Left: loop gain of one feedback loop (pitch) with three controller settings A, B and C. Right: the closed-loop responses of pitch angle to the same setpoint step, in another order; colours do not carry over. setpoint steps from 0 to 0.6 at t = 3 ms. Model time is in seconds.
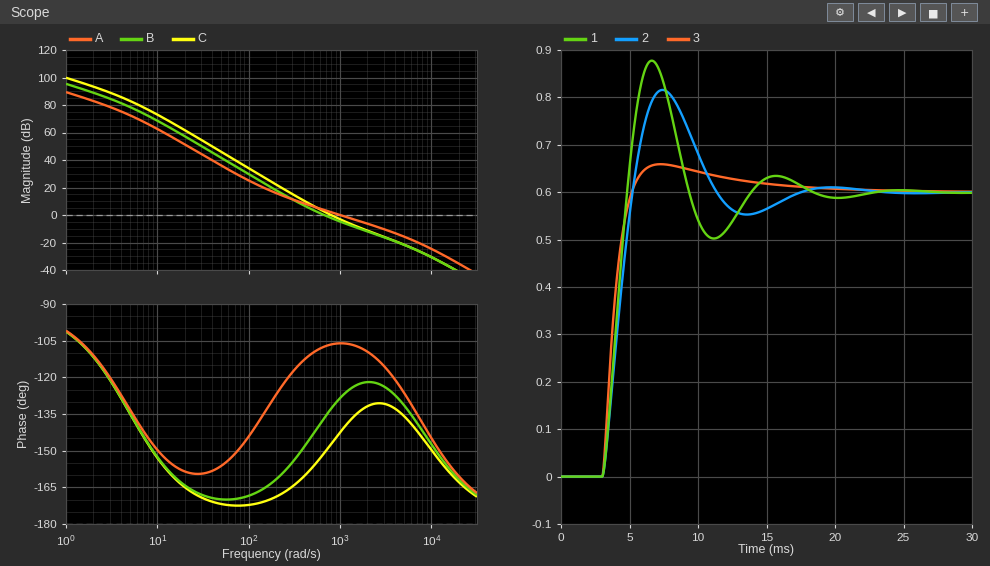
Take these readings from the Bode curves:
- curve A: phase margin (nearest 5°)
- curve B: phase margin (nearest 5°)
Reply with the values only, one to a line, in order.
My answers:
75°
45°
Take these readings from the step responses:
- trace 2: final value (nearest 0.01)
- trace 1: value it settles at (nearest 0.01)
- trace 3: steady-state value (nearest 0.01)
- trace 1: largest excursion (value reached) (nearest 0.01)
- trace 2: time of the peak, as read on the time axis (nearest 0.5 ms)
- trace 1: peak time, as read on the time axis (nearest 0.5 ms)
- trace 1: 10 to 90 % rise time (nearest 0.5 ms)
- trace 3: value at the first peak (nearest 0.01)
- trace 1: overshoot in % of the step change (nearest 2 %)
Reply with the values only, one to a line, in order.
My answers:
0.60
0.60
0.60
0.88
7.5 ms
6.5 ms
1.5 ms
0.66
46 %
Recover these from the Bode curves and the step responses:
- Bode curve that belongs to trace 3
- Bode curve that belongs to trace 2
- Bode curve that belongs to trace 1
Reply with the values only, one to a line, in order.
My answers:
A
B
C
